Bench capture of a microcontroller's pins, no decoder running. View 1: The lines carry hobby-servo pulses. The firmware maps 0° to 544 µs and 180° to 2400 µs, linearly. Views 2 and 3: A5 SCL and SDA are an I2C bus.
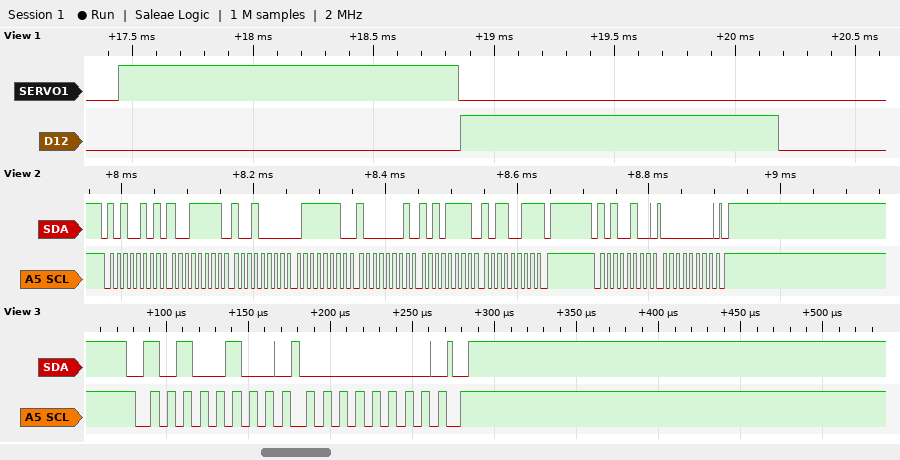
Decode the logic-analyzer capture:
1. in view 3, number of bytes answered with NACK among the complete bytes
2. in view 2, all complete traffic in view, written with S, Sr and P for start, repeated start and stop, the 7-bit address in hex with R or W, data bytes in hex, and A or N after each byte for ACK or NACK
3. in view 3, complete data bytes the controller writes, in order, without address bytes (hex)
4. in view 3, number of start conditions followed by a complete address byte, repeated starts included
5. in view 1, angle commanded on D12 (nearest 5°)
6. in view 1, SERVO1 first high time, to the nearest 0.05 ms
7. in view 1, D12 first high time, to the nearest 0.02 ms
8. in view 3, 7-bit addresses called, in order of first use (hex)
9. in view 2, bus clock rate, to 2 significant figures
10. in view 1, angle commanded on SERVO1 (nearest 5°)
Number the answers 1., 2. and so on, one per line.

1. 0
2. S 52R A 9F A 90 A 7E A 81 A AF A B3 N P S 52W A 00 A P
3. 00
4. 1
5. 75°
6. 1.40 ms
7. 1.32 ms
8. 0x52
9. 100 kHz
10. 85°
